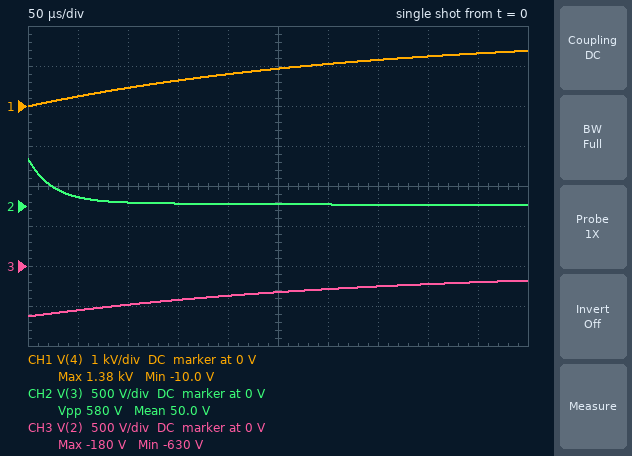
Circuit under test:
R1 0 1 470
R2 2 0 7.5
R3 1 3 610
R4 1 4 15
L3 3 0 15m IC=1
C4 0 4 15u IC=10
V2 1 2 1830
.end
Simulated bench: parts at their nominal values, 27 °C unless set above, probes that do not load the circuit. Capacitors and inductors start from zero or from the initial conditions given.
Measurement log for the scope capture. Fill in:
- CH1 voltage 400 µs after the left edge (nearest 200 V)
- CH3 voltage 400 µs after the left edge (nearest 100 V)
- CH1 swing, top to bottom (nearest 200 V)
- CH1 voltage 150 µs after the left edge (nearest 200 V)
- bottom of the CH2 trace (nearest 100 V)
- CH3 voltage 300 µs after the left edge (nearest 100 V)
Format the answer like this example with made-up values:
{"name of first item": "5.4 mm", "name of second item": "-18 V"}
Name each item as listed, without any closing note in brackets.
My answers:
{"CH1 voltage 400 µs after the left edge": "1.2 kV", "CH3 voltage 400 µs after the left edge": "-200 V", "CH1 swing, top to bottom": "1.4 kV", "CH1 voltage 150 µs after the left edge": "600 V", "bottom of the CH2 trace": "0 V", "CH3 voltage 300 µs after the left edge": "-300 V"}
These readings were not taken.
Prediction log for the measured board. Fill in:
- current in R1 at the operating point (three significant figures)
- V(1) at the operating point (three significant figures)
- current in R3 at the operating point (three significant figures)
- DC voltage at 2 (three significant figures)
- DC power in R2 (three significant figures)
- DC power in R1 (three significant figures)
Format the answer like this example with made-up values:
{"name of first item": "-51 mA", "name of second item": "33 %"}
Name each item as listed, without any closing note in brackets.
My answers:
{"current in R1 at the operating point": "3.79 A", "V(1) at the operating point": "1.78 kV", "current in R3 at the operating point": "2.92 A", "DC voltage at 2": "-50.3 V", "DC power in R2": "337 W", "DC power in R1": "6.74 kW"}
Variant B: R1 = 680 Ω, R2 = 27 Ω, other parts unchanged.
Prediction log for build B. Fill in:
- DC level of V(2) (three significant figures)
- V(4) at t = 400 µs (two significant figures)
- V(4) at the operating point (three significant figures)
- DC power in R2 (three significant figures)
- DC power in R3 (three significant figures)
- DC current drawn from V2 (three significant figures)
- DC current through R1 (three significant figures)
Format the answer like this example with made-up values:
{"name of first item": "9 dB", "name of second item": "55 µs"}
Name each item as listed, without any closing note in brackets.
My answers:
{"DC level of V(2)": "-142 V", "V(4) at t = 400 µs": "820 V", "V(4) at the operating point": "1.69 kV", "DC power in R2": "744 W", "DC power in R3": "4.67 kW", "DC current drawn from V2": "5.25 A", "DC current through R1": "2.48 A"}
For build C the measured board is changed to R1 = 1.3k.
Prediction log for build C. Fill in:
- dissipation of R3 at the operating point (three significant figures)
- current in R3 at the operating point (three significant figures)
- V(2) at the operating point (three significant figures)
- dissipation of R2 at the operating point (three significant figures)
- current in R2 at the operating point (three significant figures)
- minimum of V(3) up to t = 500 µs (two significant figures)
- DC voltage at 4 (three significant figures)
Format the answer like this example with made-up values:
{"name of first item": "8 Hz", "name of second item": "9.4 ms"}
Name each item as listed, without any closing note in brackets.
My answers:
{"dissipation of R3 at the operating point": "5.30 kW", "current in R3 at the operating point": "2.95 A", "V(2) at the operating point": "-32.5 V", "dissipation of R2 at the operating point": "141 W", "current in R2 at the operating point": "4.33 A", "minimum of V(3) up to t = 500 µs": "11 V", "DC voltage at 4": "1.80 kV"}
